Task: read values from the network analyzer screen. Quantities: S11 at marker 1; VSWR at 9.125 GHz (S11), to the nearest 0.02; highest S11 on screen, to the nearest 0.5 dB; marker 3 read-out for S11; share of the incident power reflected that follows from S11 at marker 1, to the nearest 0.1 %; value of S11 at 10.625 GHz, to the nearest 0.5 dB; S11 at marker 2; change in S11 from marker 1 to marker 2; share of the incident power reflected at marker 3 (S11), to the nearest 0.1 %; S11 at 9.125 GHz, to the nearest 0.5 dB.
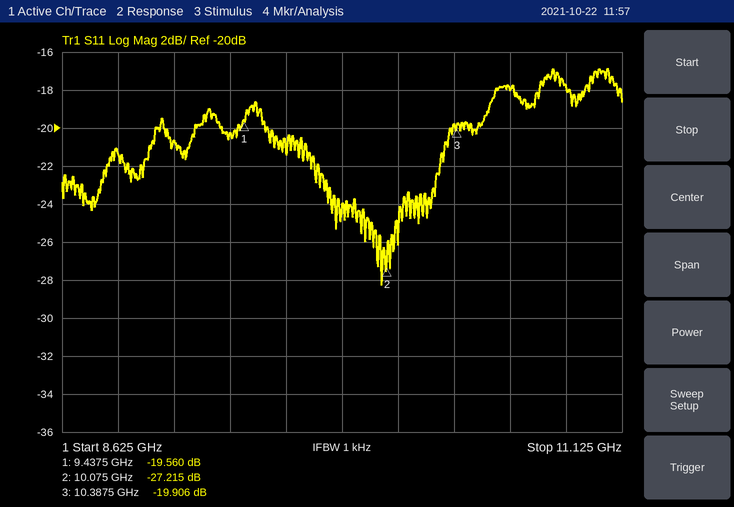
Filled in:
-19.560 dB
1.20
-17.0 dB
-19.906 dB
1.1 %
-18.0 dB
-27.215 dB
-7.655 dB
1.0 %
-20.5 dB
